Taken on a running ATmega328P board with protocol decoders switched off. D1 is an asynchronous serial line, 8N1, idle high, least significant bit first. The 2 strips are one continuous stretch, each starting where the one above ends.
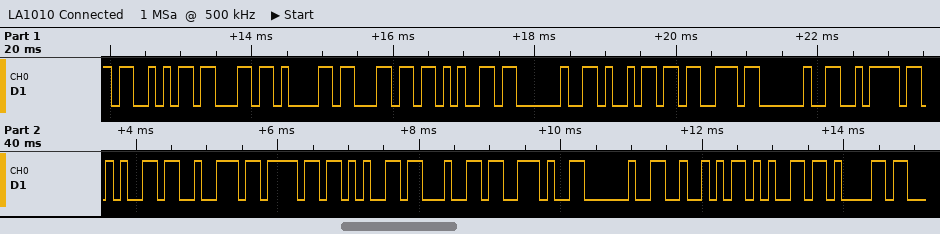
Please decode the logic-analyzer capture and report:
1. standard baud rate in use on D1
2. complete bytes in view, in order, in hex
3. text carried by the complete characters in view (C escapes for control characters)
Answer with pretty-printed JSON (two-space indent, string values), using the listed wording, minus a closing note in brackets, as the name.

{
  "standard baud rate in use on D1": "9600 baud",
  "complete bytes in view, in order, in hex": "0x53 0x63 0x61 0x6C 0x65 0x20 0x69 0x73 0x20 0x7A 0x65 0x72 0x6F 0x65 0x64 0x2E 0x20 0x52 0x65 0x61",
  "text carried by the complete characters in view": "\"Scale is zeroed. Rea\""
}
